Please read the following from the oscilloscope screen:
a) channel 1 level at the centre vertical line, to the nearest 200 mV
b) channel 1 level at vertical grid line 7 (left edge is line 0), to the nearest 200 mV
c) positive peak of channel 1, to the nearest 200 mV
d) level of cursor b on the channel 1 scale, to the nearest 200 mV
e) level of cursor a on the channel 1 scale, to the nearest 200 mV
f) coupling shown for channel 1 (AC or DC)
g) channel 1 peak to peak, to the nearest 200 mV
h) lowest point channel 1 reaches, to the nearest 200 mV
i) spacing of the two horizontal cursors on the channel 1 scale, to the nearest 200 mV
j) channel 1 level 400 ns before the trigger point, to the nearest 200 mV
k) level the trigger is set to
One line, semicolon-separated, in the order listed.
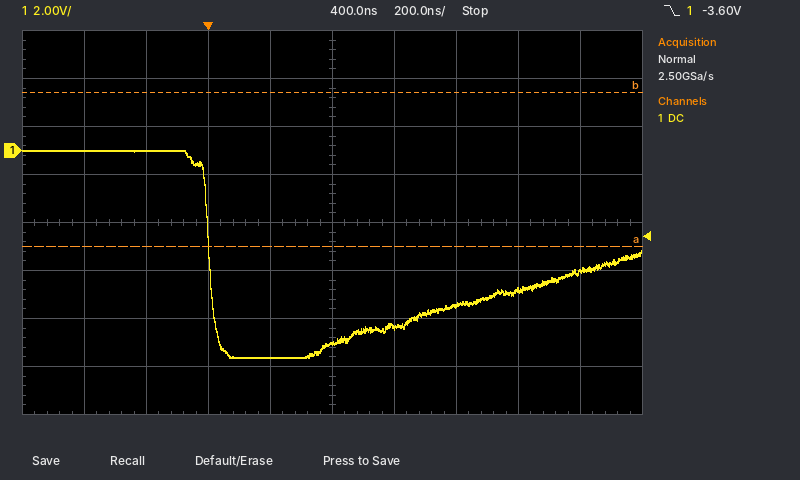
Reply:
-8.0 V; -6.4 V; 0.0 V; 2.4 V; -4.0 V; DC; 8.6 V; -8.6 V; 6.4 V; 0.0 V; -3.60 V
